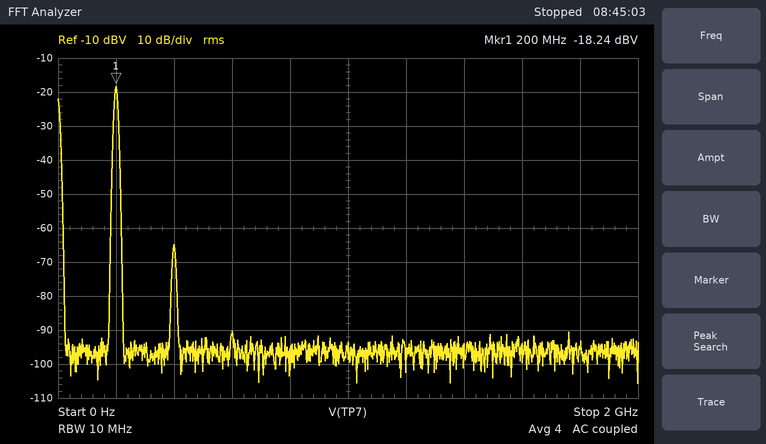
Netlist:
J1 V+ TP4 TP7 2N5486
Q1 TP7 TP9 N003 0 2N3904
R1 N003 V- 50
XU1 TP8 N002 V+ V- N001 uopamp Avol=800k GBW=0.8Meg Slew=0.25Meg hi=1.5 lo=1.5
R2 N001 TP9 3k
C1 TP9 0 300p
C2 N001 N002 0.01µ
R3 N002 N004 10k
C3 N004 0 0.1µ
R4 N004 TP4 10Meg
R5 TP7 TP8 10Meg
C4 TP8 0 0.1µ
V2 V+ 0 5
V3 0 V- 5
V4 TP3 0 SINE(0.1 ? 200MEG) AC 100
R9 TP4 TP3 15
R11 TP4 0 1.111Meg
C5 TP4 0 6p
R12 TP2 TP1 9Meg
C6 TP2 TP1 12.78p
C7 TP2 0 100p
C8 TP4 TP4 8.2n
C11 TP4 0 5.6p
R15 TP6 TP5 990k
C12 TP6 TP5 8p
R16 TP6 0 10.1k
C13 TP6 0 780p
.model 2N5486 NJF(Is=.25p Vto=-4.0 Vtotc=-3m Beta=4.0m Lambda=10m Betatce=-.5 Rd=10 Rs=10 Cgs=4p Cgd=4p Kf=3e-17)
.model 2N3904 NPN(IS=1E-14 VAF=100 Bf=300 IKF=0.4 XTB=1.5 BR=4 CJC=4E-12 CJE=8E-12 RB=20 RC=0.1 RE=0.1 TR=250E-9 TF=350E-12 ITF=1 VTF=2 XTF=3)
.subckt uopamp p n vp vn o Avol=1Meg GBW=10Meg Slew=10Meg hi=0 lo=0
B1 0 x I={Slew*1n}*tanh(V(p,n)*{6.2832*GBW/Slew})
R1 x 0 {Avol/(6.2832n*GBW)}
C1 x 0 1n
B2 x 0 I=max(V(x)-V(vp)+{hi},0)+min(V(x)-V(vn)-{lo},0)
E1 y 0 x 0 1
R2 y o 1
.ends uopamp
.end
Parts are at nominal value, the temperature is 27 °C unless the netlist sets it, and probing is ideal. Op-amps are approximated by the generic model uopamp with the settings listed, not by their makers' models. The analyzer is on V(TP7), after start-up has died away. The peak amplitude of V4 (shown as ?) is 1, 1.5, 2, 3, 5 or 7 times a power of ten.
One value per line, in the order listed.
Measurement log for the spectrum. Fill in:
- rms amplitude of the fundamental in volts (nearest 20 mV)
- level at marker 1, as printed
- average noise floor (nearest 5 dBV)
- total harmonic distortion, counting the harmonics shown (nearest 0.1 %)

120 mV
-18.24 dBV
-95 dBV
0.5 %
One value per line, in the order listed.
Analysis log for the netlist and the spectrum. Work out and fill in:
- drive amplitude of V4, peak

200 mV
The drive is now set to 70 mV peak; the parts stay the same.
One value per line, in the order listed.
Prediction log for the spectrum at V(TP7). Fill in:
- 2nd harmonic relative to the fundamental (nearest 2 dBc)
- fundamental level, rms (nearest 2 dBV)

-56 dBc
-28 dBV
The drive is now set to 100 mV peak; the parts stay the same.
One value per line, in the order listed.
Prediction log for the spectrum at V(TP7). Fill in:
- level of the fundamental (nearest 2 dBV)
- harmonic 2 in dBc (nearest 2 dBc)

-24 dBV
-52 dBc
